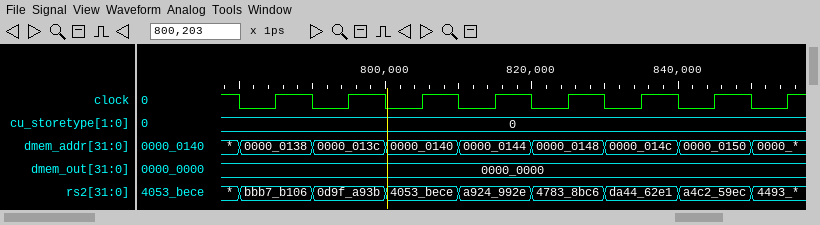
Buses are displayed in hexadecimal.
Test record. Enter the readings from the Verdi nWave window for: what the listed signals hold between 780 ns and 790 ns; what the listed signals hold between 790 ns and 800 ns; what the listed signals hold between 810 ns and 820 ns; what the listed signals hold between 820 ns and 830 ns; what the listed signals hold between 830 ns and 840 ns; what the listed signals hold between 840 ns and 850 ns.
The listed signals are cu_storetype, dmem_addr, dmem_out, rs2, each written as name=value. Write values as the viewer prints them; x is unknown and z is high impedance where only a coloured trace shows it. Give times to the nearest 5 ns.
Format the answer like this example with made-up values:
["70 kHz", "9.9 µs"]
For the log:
["cu_storetype=0, dmem_addr=0000_0138, dmem_out=0000_0000, rs2=bbb7_b106", "cu_storetype=0, dmem_addr=0000_013c, dmem_out=0000_0000, rs2=0d9f_a93b", "cu_storetype=0, dmem_addr=0000_0144, dmem_out=0000_0000, rs2=a924_992e", "cu_storetype=0, dmem_addr=0000_0148, dmem_out=0000_0000, rs2=4783_8bc6", "cu_storetype=0, dmem_addr=0000_014c, dmem_out=0000_0000, rs2=da44_62e1", "cu_storetype=0, dmem_addr=0000_0150, dmem_out=0000_0000, rs2=a4c2_59ec"]
